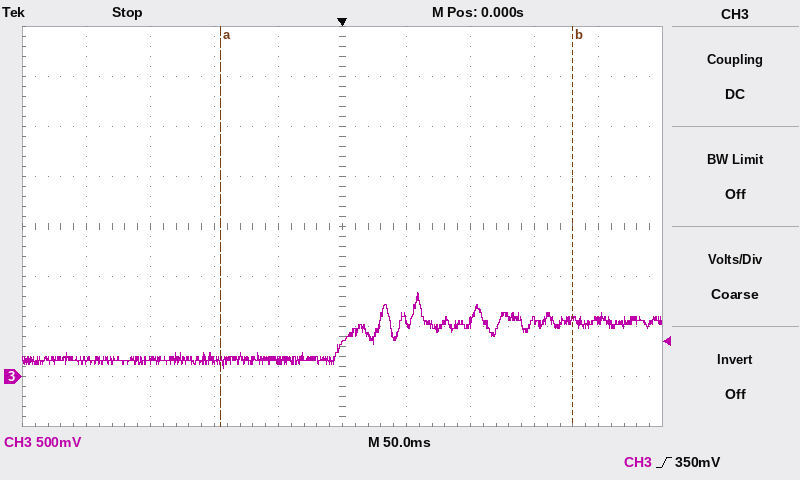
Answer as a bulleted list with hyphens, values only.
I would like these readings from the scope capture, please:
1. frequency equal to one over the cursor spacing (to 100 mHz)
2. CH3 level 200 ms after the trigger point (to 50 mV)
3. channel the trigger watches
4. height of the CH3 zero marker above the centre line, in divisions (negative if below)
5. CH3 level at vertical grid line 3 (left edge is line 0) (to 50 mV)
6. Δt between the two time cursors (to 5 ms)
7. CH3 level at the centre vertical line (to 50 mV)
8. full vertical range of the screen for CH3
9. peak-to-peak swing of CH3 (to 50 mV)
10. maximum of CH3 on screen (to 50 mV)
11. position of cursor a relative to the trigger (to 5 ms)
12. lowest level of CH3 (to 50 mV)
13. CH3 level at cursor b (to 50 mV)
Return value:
- 3.6 Hz
- 550 mV
- CH3
- -3.0 div
- 150 mV
- 275 ms
- 300 mV
- 4 V
- 750 mV
- 850 mV
- -95 ms
- 100 mV
- 550 mV
